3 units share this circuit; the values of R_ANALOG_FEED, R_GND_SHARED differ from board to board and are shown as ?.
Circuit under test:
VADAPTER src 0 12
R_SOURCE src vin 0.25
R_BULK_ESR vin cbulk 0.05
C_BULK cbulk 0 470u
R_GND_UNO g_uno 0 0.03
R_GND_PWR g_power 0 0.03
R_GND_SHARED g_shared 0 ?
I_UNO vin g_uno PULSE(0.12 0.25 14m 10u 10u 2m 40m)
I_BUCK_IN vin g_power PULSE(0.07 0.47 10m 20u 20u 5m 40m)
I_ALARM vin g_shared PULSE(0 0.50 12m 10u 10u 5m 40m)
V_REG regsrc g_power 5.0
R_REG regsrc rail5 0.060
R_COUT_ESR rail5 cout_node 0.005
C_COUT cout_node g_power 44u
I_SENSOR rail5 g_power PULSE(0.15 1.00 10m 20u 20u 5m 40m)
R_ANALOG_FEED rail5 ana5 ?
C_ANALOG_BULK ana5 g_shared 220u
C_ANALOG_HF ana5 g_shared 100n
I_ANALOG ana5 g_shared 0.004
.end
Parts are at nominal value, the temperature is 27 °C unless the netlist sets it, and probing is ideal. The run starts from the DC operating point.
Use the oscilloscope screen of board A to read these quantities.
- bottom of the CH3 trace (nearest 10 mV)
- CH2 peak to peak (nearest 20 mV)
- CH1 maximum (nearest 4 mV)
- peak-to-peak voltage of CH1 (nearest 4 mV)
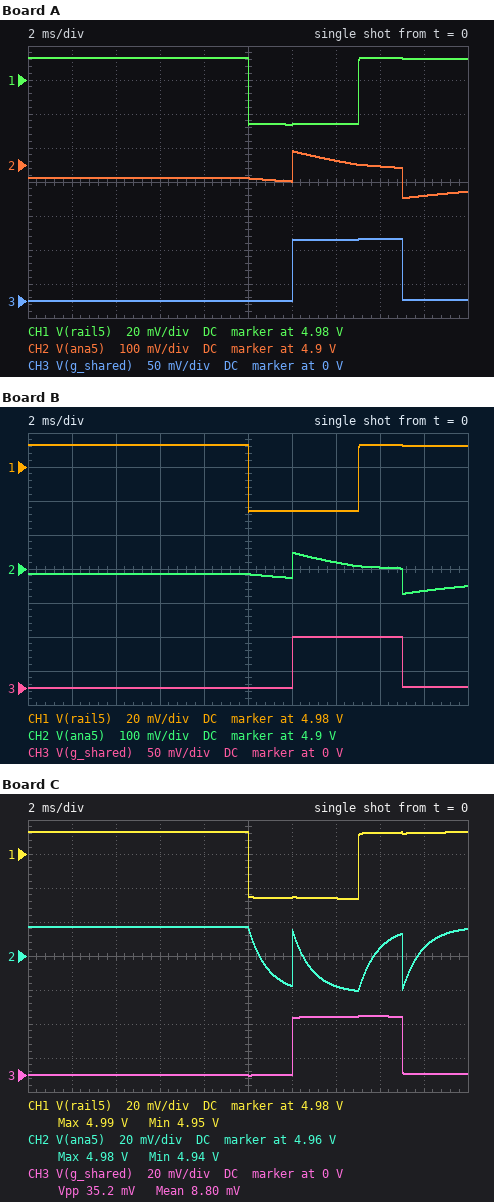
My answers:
0 V
140 mV
4.992 V
40 mV
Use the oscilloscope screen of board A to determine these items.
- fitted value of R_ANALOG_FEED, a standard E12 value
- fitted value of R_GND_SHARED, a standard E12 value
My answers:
33 Ω
0.18 Ω
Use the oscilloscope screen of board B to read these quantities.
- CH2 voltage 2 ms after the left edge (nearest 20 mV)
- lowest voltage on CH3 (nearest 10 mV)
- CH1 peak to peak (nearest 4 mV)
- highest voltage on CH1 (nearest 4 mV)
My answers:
4.88 V
0 V
40 mV
4.992 V
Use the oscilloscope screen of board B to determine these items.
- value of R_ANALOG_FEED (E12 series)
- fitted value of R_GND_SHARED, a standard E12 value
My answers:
27 Ω
0.15 Ω
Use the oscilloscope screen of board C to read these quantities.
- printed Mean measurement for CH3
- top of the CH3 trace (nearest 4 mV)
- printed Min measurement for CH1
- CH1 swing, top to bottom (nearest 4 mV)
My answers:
8.80 mV
36 mV
4.95 V
40 mV
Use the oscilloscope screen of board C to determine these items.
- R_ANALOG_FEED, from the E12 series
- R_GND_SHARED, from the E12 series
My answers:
3.9 Ω
0.068 Ω
